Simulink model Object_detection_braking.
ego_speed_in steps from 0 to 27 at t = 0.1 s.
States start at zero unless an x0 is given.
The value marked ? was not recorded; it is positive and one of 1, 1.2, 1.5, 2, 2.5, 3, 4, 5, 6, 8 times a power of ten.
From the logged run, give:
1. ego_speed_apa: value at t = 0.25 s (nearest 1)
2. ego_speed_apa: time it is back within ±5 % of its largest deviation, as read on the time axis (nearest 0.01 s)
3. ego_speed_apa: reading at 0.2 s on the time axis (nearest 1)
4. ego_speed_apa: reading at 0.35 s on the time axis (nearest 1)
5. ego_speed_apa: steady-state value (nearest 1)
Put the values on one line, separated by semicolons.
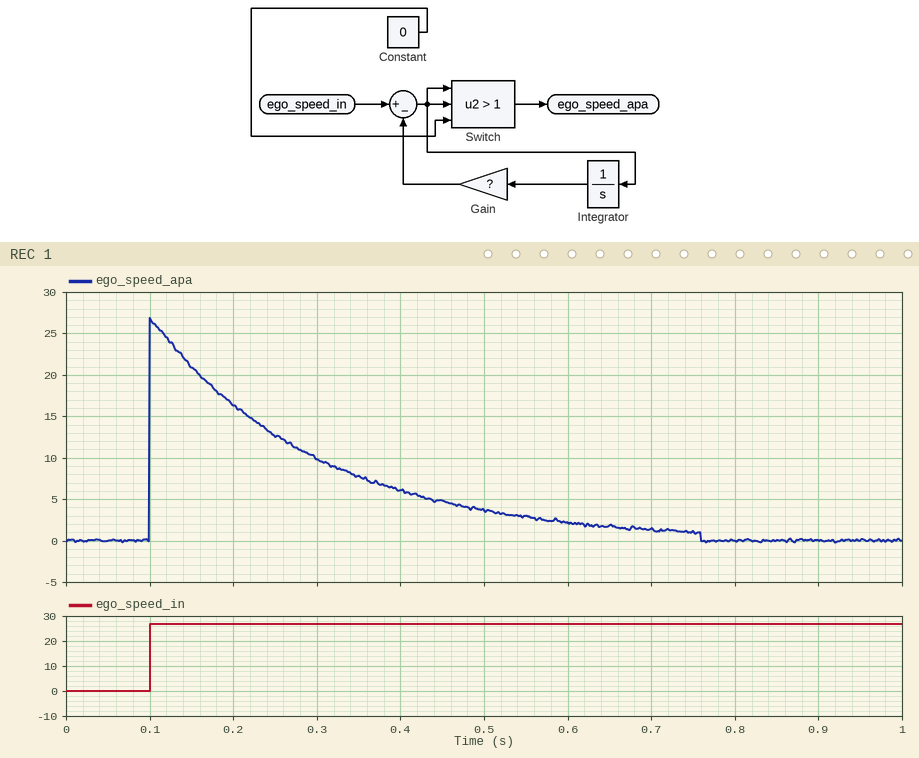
13; 0.70 s; 16; 8; 0
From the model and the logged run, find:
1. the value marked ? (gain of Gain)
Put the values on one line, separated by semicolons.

5
